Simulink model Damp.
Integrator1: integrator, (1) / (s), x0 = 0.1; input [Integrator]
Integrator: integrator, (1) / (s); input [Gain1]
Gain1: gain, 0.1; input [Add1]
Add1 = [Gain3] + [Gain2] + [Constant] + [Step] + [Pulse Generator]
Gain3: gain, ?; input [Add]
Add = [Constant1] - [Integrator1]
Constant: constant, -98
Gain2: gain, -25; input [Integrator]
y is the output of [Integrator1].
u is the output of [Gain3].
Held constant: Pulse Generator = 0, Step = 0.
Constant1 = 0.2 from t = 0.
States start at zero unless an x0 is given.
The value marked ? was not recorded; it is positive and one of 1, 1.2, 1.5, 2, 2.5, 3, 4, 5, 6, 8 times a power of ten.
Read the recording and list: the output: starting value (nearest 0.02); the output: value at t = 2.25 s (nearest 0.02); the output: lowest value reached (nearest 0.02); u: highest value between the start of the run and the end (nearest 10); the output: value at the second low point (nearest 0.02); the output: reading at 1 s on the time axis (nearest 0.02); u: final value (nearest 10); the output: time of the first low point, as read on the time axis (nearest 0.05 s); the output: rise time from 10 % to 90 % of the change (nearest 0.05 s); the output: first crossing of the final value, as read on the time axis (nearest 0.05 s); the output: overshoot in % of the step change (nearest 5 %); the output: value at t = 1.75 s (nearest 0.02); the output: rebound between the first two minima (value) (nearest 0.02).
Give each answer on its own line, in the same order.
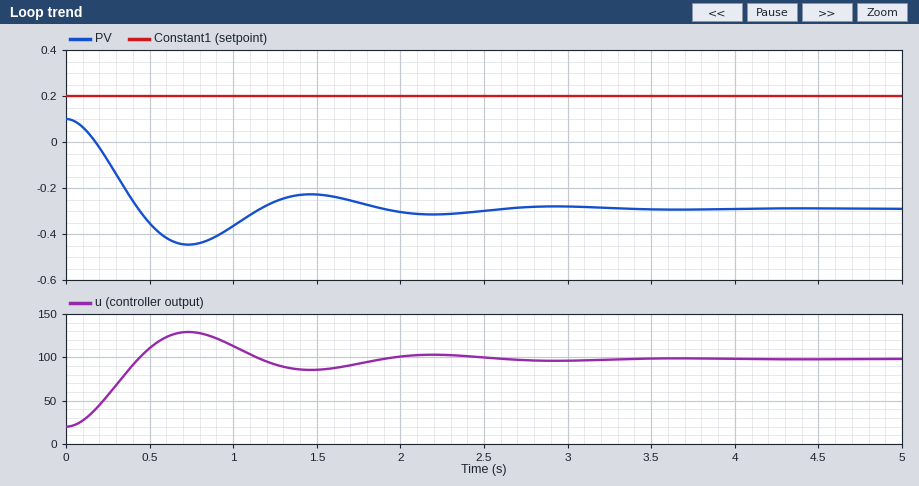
0.10
-0.32
-0.44
130
-0.32
-0.36
100
0.75 s
0.30 s
0.45 s
40 %
-0.26
-0.22
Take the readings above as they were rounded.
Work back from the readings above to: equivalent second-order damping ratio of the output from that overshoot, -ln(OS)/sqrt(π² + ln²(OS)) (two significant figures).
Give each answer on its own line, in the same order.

0.28
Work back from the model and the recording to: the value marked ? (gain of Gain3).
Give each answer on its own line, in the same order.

200
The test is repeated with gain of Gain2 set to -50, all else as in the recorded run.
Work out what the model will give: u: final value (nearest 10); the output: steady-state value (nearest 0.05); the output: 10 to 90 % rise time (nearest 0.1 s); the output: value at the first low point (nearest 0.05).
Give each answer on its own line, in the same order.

100
-0.30
0.4 s
-0.35
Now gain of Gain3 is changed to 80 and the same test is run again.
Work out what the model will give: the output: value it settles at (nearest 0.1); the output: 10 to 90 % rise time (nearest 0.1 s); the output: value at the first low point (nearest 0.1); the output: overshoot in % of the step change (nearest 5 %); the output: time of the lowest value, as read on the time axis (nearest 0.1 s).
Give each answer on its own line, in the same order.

-1.0
0.5 s
-1.3
20 %
1.2 s
